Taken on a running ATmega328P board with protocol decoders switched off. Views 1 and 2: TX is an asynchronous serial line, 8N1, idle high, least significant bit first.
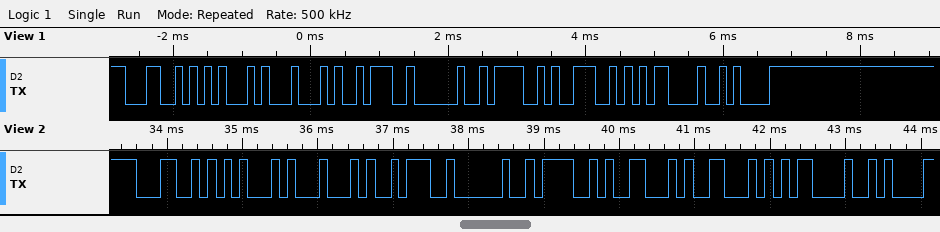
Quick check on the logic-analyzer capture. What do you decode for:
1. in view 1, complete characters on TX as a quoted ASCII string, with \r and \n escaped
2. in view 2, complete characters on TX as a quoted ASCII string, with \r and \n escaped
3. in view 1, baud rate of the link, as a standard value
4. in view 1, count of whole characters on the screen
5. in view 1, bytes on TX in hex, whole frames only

"LED: ON\r\n"
"LED: OFF\r\n"
9600 baud
9
0x4C 0x45 0x44 0x3A 0x20 0x4F 0x4E 0x0D 0x0A
